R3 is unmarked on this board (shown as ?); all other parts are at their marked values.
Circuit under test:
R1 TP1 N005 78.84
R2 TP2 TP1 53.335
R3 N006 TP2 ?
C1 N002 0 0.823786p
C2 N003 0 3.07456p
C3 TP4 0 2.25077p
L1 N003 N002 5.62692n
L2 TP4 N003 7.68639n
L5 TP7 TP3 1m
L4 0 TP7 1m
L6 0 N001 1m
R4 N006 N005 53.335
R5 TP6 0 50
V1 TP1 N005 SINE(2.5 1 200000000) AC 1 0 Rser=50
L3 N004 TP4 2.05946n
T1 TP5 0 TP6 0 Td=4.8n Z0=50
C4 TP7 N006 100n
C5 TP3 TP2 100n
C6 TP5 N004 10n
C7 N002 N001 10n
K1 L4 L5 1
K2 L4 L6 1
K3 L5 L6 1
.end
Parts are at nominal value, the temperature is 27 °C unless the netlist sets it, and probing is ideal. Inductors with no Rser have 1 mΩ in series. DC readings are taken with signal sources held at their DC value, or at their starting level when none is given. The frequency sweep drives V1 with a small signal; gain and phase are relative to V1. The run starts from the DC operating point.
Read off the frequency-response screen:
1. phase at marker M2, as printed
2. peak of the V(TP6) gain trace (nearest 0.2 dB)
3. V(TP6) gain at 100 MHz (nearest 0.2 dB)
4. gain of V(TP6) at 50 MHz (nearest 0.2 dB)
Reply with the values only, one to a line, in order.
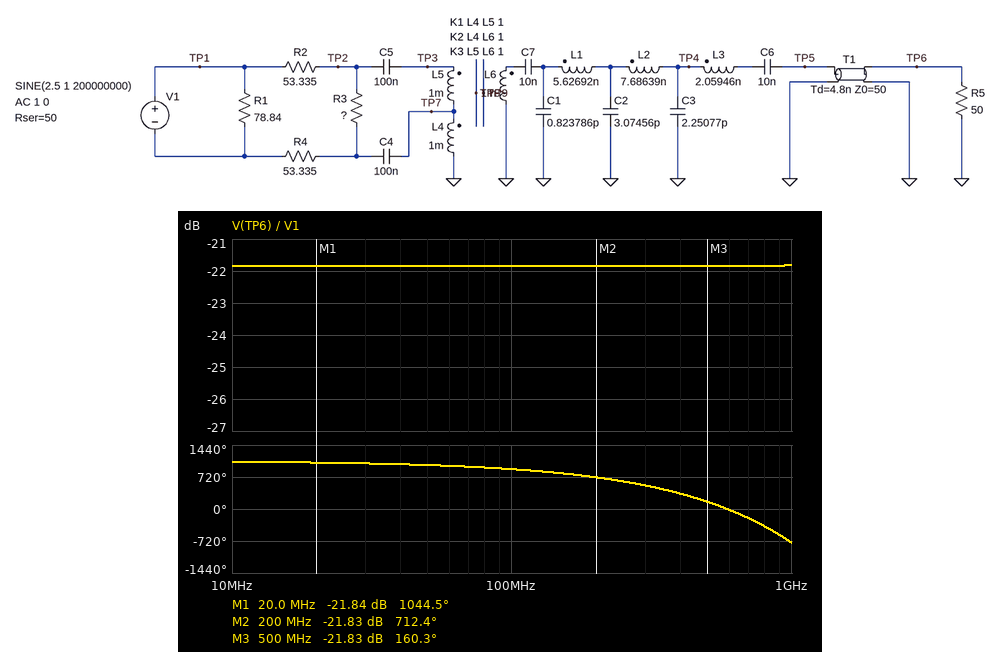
712.4 deg
-21.8 dB
-21.8 dB
-21.8 dB
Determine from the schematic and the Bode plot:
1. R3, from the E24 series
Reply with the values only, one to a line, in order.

36 Ω
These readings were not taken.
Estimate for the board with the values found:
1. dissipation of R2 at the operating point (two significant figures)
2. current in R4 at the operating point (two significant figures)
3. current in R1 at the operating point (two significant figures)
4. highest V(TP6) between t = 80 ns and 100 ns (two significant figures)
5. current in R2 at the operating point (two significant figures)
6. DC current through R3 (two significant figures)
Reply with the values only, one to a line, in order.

4.2 mW
8.8 mA
16 mA
81 mV
8.8 mA
8.8 mA
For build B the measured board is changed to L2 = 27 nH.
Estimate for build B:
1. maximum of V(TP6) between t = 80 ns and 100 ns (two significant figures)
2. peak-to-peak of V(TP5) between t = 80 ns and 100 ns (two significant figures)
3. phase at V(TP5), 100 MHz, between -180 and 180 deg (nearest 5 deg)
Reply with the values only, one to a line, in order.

75 mV
150 mV
-20 deg
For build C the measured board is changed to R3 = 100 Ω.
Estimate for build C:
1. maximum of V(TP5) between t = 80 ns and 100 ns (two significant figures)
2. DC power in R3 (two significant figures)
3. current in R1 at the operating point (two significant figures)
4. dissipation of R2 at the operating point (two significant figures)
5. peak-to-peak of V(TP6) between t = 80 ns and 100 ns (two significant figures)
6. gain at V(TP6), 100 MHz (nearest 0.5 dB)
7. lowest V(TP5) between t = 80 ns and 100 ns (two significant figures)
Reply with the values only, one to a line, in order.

120 mV
4.2 mW
17 mA
2.2 mW
240 mV
-18.5 dB
-120 mV
